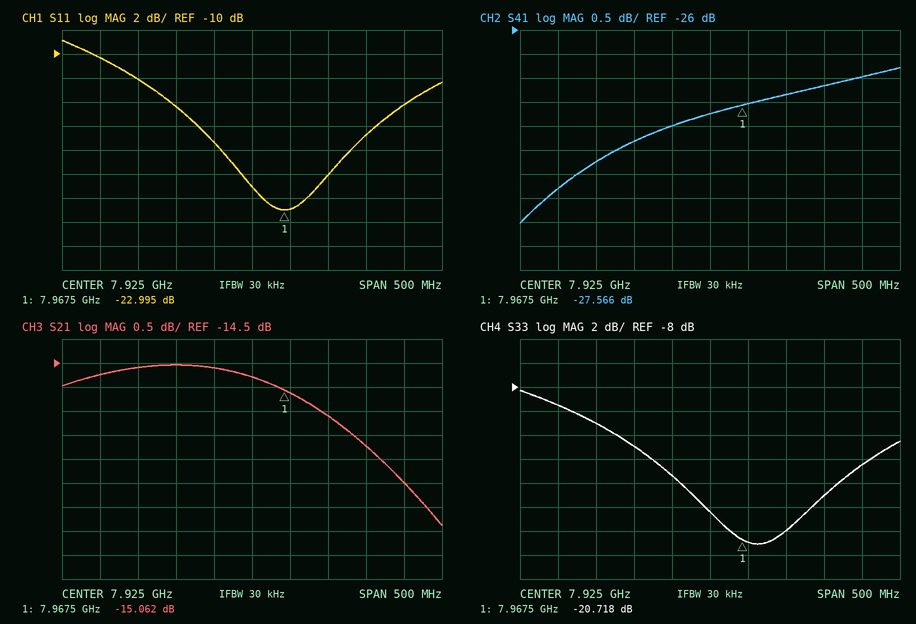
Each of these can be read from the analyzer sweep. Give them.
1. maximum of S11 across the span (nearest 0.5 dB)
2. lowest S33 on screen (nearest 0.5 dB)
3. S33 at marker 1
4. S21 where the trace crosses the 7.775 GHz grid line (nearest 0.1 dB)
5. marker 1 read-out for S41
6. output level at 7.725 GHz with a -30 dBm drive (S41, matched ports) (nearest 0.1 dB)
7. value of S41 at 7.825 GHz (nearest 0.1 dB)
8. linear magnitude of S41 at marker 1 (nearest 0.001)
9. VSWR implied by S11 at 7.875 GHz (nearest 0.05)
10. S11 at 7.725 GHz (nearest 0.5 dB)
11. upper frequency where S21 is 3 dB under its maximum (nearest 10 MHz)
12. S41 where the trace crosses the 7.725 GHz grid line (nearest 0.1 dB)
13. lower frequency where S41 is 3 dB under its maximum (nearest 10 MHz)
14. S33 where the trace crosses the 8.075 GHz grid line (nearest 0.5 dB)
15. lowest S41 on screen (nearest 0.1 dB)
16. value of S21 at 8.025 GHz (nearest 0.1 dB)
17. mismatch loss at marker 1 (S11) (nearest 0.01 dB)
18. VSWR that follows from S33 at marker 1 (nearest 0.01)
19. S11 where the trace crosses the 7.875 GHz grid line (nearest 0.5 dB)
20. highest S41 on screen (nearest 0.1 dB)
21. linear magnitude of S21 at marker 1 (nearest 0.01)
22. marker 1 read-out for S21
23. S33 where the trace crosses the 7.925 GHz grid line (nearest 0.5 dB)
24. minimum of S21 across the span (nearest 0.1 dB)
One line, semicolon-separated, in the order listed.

-9.0 dB; -21.0 dB; -20.718 dB; -14.6 dB; -27.566 dB; -59.3 dBm; -28.3 dB; 0.042; 1.30; -10.5 dB; 8.16 GHz; -29.3 dB; 7.69 GHz; -17.0 dB; -30.0 dB; -15.6 dB; 0.02 dB; 1.20; -17.5 dB; -26.8 dB; 0.18; -15.062 dB; -18.5 dB; -17.9 dB
